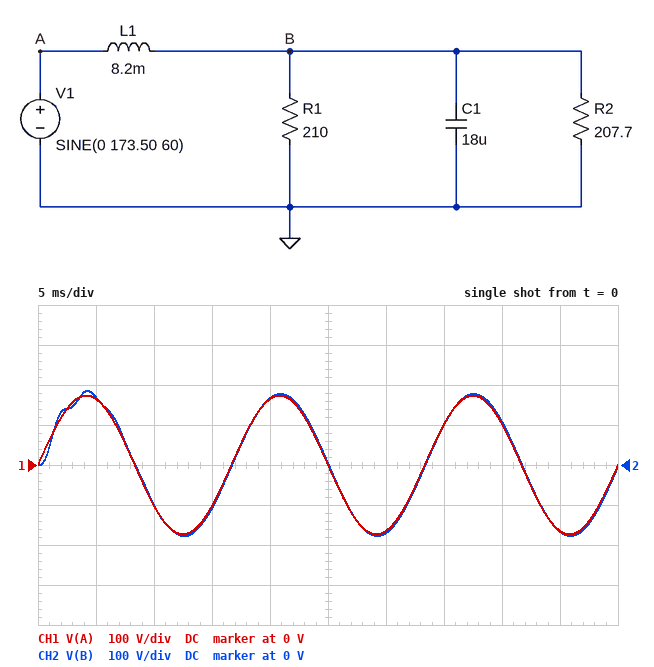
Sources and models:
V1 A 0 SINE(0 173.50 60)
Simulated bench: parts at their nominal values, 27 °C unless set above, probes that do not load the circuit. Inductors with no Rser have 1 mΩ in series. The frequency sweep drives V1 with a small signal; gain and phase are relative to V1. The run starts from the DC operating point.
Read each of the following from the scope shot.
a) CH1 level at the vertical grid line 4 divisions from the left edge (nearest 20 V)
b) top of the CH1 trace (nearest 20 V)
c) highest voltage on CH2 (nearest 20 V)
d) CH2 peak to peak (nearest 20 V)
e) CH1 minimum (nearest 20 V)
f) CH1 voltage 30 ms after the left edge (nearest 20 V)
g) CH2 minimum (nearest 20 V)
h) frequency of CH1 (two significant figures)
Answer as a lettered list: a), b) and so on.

a) 160 V
b) 180 V
c) 180 V
d) 360 V
e) -180 V
f) -160 V
g) -180 V
h) 60 Hz
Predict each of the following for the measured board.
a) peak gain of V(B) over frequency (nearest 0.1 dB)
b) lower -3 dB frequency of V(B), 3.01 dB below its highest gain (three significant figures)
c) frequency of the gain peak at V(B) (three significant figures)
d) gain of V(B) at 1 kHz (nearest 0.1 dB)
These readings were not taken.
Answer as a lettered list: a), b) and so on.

a) 13.8 dB
b) 365 Hz
c) 410 Hz
d) -13.7 dB
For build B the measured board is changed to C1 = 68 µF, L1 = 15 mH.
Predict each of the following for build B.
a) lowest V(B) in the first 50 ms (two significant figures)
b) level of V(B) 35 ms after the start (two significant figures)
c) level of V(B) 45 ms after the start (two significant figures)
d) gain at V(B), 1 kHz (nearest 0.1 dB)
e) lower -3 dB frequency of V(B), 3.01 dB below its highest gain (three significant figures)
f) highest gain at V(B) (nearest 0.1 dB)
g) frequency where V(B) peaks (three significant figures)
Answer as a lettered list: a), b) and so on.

a) -210 V
b) 110 V
c) -190 V
d) -31.9 dB
e) 145 Hz
f) 17.0 dB
g) 157 Hz
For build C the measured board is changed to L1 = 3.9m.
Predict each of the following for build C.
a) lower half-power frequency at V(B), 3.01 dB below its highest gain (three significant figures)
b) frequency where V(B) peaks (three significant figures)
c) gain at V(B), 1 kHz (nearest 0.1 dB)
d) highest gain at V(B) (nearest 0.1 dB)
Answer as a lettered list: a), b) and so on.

a) 554 Hz
b) 598 Hz
c) -5.0 dB
d) 17.0 dB
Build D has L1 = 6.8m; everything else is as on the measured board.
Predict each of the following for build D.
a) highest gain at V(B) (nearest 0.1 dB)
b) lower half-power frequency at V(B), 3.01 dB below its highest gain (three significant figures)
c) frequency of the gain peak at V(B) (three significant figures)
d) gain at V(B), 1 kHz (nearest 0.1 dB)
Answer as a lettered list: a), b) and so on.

a) 14.6 dB
b) 406 Hz
c) 451 Hz
d) -11.7 dB
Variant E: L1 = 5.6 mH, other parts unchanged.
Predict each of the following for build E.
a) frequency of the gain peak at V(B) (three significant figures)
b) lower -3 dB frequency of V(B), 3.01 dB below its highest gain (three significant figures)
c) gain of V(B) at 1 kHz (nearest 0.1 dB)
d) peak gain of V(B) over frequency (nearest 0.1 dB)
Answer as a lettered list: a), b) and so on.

a) 498 Hz
b) 453 Hz
c) -9.5 dB
d) 15.5 dB
